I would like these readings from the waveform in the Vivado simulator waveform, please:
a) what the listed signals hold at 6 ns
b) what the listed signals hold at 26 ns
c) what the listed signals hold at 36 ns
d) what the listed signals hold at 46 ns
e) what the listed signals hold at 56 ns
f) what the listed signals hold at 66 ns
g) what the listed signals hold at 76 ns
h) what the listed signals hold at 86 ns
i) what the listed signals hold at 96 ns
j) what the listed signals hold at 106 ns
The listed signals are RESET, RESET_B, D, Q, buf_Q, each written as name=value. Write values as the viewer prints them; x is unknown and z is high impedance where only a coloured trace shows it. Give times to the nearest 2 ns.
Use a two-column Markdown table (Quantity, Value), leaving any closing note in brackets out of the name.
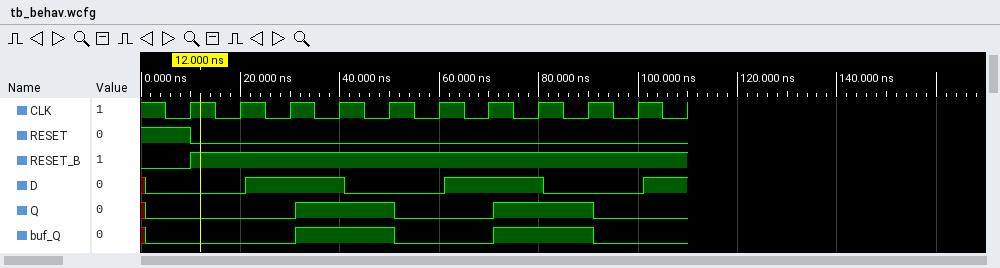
| Quantity | Value |
|---|---|
| what the listed signals hold at 6 ns | RESET=1, RESET_B=0, D=0, Q=0, buf_Q=0 |
| what the listed signals hold at 26 ns | RESET=0, RESET_B=1, D=1, Q=0, buf_Q=0 |
| what the listed signals hold at 36 ns | RESET=0, RESET_B=1, D=1, Q=1, buf_Q=1 |
| what the listed signals hold at 46 ns | RESET=0, RESET_B=1, D=0, Q=1, buf_Q=1 |
| what the listed signals hold at 56 ns | RESET=0, RESET_B=1, D=0, Q=0, buf_Q=0 |
| what the listed signals hold at 66 ns | RESET=0, RESET_B=1, D=1, Q=0, buf_Q=0 |
| what the listed signals hold at 76 ns | RESET=0, RESET_B=1, D=1, Q=1, buf_Q=1 |
| what the listed signals hold at 86 ns | RESET=0, RESET_B=1, D=0, Q=1, buf_Q=1 |
| what the listed signals hold at 96 ns | RESET=0, RESET_B=1, D=0, Q=0, buf_Q=0 |
| what the listed signals hold at 106 ns | RESET=0, RESET_B=1, D=1, Q=0, buf_Q=0 |
